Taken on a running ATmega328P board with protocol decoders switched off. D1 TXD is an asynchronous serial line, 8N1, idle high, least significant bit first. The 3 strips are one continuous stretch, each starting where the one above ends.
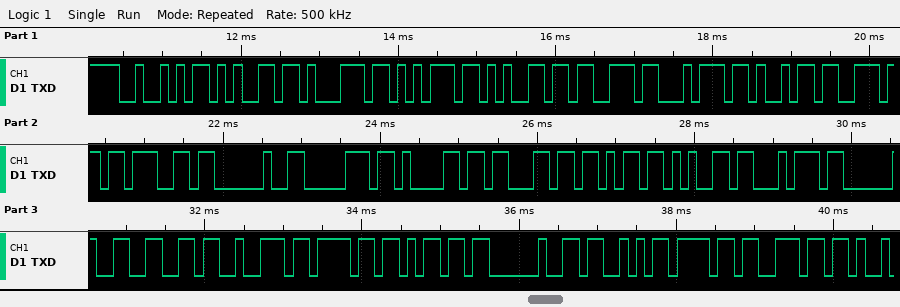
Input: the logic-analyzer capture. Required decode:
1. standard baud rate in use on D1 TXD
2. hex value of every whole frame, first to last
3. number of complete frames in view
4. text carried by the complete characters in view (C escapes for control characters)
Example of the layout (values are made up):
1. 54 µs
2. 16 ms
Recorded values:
1. 9600 baud
2. 52 65 71 75 65 73 74 69 6E 67 20 70 61 63 6B 65 74 20 66 72 6F 6D 20 53 6F 6E
3. 26
4. "Requesting packet from Son"
